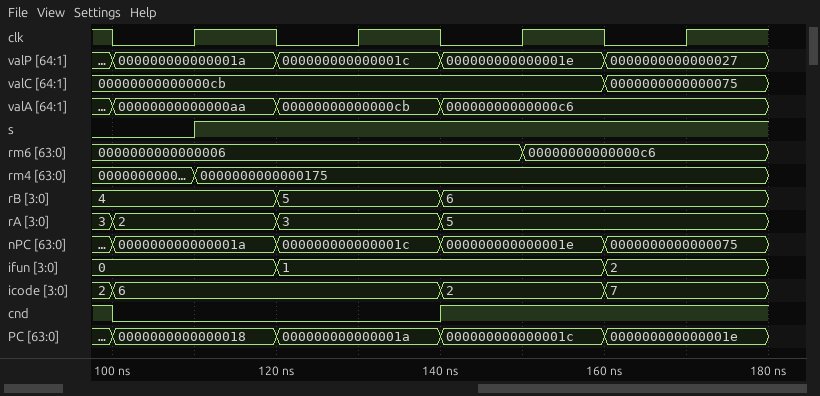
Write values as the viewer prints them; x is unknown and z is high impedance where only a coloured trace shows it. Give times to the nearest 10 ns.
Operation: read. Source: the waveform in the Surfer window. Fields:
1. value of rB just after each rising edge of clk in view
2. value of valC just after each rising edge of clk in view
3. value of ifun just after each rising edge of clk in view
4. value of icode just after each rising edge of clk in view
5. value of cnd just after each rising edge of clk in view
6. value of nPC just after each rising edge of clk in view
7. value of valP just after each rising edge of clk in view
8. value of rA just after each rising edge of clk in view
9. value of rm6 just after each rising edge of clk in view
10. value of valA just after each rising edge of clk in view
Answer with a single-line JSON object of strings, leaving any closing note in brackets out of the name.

{"value of rB just after each rising edge of clk in view": "4, 5, 6, 6", "value of valC just after each rising edge of clk in view": "00000000000000cb, 00000000000000cb, 00000000000000cb, 0000000000000075", "value of ifun just after each rising edge of clk in view": "0, 1, 1, 2", "value of icode just after each rising edge of clk in view": "6, 6, 2, 7", "value of cnd just after each rising edge of clk in view": "0 0 1 1", "value of nPC just after each rising edge of clk in view": "000000000000001a, 000000000000001c, 000000000000001e, 0000000000000075", "value of valP just after each rising edge of clk in view": "000000000000001a, 000000000000001c, 000000000000001e, 0000000000000027", "value of rA just after each rising edge of clk in view": "2, 3, 5, 5", "value of rm6 just after each rising edge of clk in view": "0000000000000006, 0000000000000006, 00000000000000c6, 00000000000000c6", "value of valA just after each rising edge of clk in view": "00000000000000aa, 00000000000000cb, 00000000000000c6, 00000000000000c6"}
